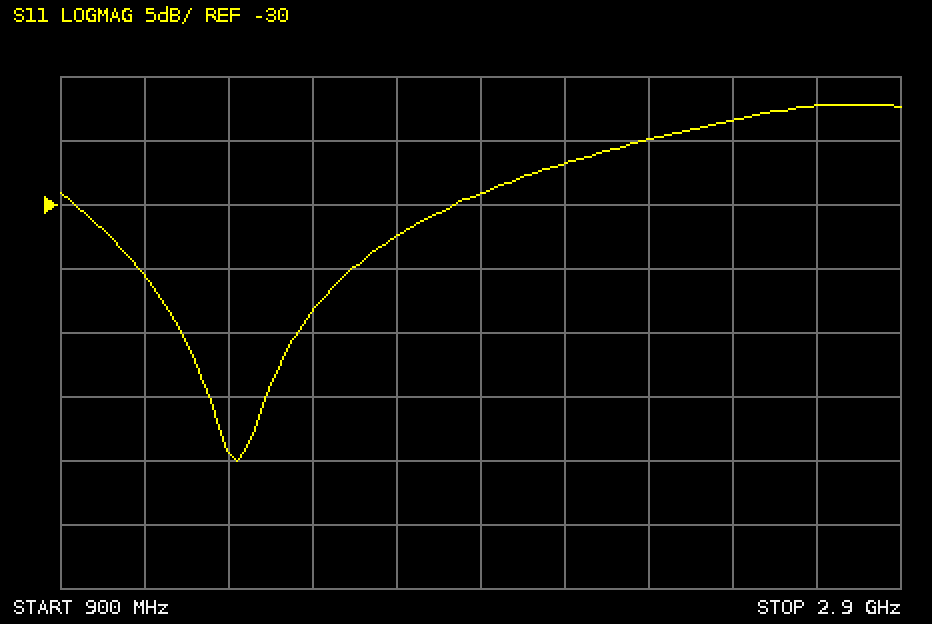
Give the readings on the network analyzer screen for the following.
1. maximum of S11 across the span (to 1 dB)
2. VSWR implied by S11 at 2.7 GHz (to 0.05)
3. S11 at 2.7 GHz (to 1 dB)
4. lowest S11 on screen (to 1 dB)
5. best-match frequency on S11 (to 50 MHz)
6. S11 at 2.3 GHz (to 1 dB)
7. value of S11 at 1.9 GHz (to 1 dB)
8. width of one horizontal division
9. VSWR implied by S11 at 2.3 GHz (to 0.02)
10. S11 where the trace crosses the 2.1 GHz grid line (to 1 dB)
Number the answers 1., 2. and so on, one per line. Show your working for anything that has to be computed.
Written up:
1. -22 dB
2. |Γ| = 10^(-22/20) = 0.0794; VSWR = (1 + 0.0794)/(1 − 0.0794) ≈ 1.17, so 1.15 to the nearest 0.05
3. -22 dB
4. -50 dB
5. 1.30 GHz
6. -25 dB
7. -29 dB
8. 200 MHz
9. |Γ| = 10^(-25/20) = 0.0562; VSWR = (1 + 0.0562)/(1 − 0.0562) ≈ 1.12
10. -27 dB
